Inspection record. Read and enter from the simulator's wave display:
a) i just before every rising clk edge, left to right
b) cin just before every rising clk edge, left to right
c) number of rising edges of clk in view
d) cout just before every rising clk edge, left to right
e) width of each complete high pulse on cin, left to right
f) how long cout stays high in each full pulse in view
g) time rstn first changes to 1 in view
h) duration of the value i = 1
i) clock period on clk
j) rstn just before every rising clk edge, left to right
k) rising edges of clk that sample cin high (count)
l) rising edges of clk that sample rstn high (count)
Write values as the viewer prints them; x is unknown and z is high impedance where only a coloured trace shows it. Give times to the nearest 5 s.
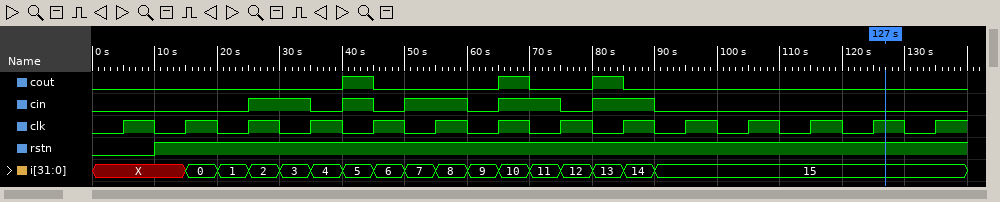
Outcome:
X, X, 1, 3, 5, 7, 9, 11, 13, 15, 15, 15, 15, 15
0 0 0 1 1 1 0 1 1 0 0 0 0 0
14
0 0 0 0 1 0 0 0 1 0 0 0 0 0
10 s, 5 s, 10 s, 10 s, 10 s
5 s, 5 s, 5 s
10 s
5 s
10 s
0 1 1 1 1 1 1 1 1 1 1 1 1 1
5
13
